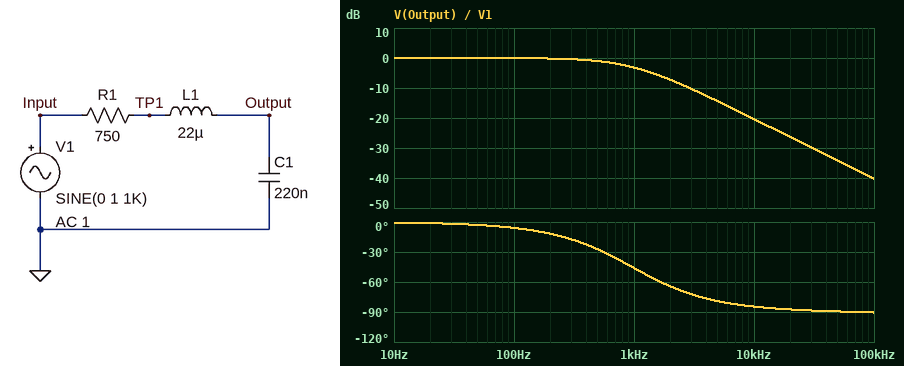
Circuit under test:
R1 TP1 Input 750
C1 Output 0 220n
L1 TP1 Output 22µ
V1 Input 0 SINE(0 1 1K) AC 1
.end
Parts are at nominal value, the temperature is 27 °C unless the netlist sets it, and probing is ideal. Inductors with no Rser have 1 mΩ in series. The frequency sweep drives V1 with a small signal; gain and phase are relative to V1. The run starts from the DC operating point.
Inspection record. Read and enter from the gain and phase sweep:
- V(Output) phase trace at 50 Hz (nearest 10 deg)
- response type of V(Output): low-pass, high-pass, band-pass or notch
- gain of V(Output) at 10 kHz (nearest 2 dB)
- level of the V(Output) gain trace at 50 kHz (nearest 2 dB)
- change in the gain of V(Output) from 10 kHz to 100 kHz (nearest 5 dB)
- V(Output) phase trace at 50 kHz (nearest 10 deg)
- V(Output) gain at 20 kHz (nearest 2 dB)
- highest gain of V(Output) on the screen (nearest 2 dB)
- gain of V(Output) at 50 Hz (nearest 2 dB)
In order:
0 deg
low-pass
-20 dB
-34 dB
-20 dB
-90 deg
-26 dB
0 dB
0 dB
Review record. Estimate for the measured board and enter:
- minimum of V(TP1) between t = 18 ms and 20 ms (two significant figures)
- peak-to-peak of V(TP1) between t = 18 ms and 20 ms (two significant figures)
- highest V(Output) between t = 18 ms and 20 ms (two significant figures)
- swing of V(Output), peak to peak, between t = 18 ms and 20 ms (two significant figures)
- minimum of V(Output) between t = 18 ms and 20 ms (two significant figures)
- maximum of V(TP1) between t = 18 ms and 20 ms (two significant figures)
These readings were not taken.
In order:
-690 mV
1.4 V
690 mV
1.4 V
-690 mV
690 mV
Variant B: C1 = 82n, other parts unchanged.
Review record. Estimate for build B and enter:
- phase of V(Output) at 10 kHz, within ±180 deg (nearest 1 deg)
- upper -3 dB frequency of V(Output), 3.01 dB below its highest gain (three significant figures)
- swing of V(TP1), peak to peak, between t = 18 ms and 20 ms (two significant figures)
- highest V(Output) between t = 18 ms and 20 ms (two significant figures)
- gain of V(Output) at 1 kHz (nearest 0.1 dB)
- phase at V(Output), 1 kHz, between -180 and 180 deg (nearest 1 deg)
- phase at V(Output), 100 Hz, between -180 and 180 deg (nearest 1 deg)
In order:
-76 deg
2.59 kHz
1.9 V
930 mV
-0.6 dB
-21 deg
-2 deg
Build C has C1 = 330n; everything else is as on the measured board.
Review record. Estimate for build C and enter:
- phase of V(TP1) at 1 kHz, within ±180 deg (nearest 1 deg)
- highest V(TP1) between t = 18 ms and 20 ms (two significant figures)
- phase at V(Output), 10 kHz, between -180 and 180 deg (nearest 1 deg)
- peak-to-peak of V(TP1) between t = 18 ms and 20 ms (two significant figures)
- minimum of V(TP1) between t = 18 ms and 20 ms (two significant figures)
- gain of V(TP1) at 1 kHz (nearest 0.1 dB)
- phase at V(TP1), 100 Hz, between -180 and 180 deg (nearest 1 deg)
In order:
-57 deg
540 mV
-86 deg
1.1 V
-540 mV
-5.3 dB
-9 deg
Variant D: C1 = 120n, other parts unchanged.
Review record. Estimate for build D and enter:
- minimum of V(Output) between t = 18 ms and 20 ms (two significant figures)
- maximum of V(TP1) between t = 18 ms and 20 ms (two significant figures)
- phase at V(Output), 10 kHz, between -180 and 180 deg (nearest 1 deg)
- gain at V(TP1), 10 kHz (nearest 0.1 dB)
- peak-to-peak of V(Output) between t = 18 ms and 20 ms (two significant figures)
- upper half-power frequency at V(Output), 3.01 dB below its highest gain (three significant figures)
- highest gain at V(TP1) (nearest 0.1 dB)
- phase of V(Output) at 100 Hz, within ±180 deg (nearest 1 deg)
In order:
-870 mV
870 mV
-80 deg
-15.3 dB
1.7 V
1.77 kHz
0 dB
-3 deg
